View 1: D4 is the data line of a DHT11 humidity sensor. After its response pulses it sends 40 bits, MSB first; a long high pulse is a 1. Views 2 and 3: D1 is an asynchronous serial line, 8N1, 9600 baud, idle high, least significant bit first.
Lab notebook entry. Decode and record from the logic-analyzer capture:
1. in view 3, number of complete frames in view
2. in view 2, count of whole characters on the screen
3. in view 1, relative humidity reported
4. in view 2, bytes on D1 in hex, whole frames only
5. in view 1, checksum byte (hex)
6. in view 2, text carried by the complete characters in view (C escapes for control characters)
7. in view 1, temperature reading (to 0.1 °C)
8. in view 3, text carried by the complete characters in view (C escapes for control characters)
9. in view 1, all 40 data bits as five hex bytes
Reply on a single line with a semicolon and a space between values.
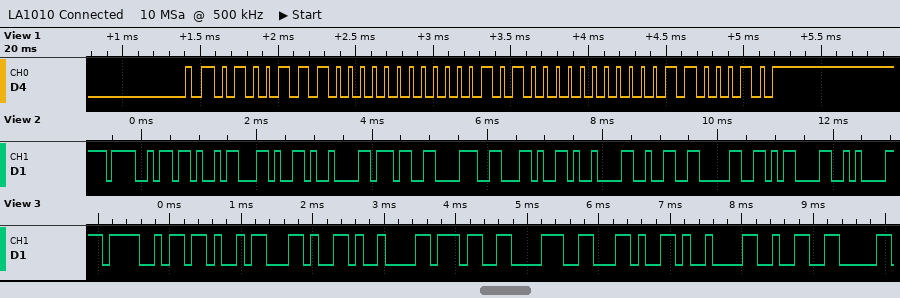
9; 12; 78 %; 4F 4B 2C 09 37 38 2C 09 32 30 0D 0A; 0x62; "OK,\t78,\t20\r\n"; 20.0 °C; "OK,\t78,\t2"; 4E 00 14 00 62
